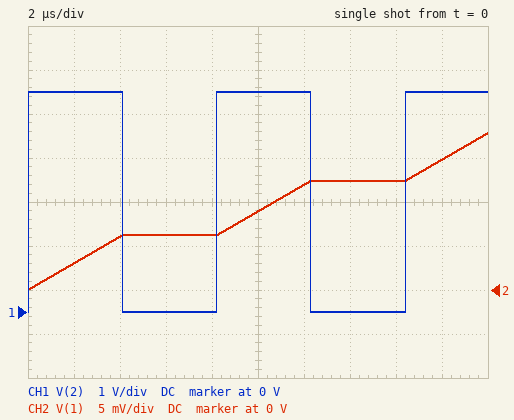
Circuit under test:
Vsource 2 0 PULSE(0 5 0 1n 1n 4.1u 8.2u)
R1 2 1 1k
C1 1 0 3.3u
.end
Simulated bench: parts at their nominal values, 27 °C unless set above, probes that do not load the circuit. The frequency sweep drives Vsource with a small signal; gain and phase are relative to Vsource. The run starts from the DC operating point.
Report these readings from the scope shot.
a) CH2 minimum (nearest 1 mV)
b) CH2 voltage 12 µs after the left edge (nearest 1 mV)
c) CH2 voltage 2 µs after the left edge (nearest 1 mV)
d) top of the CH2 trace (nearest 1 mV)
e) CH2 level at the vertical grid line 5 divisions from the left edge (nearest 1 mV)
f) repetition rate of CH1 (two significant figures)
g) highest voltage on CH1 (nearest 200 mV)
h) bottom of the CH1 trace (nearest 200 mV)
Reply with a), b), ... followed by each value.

a) 0 V
b) 12 mV
c) 3 mV
d) 18 mV
e) 9 mV
f) 120 kHz
g) 5.0 V
h) 0 V
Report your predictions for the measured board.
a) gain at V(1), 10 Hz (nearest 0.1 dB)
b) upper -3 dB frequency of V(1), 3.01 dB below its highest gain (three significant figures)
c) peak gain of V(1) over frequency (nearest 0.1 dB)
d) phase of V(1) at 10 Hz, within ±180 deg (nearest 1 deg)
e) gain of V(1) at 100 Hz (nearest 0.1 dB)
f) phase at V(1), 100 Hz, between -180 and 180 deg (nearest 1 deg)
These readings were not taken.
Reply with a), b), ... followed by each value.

a) -0.2 dB
b) 48.2 Hz
c) 0 dB
d) -12 deg
e) -7.2 dB
f) -64 deg
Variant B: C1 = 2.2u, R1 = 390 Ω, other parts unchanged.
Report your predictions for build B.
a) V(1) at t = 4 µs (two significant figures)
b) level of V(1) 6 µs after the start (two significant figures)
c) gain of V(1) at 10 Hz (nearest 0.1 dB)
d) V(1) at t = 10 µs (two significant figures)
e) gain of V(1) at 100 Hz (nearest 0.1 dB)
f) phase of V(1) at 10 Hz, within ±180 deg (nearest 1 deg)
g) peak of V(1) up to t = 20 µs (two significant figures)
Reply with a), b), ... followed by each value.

a) 23 mV
b) 24 mV
c) 0 dB
d) 34 mV
e) -1.1 dB
f) -3 deg
g) 68 mV
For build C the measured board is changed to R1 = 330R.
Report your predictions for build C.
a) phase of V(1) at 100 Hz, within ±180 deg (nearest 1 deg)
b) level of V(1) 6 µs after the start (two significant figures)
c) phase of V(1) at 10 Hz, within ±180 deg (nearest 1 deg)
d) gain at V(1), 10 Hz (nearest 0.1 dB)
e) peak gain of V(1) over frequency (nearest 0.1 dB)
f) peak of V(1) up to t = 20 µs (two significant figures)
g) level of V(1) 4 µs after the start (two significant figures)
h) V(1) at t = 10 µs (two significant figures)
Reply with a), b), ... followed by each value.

a) -34 deg
b) 19 mV
c) -4 deg
d) 0 dB
e) 0 dB
f) 54 mV
g) 18 mV
h) 27 mV
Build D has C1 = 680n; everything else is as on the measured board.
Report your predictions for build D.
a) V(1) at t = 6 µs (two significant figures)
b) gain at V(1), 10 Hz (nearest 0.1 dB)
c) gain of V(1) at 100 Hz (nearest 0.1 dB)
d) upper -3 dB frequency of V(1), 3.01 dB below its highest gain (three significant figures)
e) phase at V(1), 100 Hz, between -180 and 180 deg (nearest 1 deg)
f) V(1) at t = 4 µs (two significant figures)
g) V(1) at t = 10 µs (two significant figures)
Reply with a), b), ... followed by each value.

a) 30 mV
b) 0 dB
c) -0.7 dB
d) 234 Hz
e) -23 deg
f) 29 mV
g) 43 mV
